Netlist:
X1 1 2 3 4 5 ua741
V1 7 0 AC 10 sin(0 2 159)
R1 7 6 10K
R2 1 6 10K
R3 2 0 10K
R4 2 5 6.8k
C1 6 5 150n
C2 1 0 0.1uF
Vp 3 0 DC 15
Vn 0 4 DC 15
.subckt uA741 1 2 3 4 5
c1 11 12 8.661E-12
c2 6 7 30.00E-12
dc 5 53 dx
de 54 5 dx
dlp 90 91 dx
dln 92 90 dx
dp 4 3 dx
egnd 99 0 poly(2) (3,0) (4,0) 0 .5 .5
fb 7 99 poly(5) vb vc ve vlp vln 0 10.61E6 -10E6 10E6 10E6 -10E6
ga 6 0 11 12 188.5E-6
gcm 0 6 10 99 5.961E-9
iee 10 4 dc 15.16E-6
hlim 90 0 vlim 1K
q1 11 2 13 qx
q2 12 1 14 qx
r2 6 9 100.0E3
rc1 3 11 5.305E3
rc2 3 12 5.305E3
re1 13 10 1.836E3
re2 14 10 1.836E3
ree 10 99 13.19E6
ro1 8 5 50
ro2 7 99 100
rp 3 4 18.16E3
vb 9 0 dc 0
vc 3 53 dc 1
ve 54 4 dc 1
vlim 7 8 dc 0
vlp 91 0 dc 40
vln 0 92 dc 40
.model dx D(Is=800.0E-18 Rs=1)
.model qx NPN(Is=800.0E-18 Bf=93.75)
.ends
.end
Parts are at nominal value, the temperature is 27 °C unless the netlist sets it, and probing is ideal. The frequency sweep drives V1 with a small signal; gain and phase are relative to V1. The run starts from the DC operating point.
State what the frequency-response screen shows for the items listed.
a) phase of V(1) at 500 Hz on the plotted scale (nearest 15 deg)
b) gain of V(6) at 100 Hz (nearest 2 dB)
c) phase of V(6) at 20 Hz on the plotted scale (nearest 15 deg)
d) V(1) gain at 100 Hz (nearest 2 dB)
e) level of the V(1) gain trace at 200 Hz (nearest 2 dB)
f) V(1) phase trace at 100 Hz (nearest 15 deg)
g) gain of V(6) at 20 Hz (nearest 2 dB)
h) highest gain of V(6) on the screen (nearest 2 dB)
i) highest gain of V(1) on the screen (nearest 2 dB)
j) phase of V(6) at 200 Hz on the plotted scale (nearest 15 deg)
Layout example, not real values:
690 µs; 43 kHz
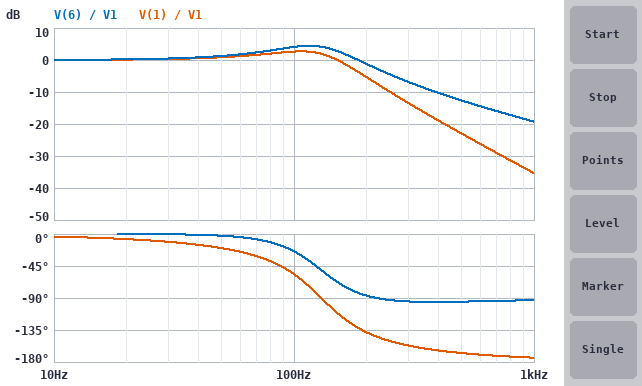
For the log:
-165 deg; 4 dB; 0 deg; 2 dB; -6 dB; -60 deg; 0 dB; 4 dB; 2 dB; -90 deg
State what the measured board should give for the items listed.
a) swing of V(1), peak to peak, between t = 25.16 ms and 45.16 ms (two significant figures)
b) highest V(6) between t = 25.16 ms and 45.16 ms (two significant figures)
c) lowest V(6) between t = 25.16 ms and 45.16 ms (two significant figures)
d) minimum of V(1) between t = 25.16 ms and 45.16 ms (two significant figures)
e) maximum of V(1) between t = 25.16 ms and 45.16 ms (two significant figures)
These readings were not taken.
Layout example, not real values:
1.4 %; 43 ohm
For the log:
3.6 V; 2.6 V; -2.6 V; -1.8 V; 1.8 V
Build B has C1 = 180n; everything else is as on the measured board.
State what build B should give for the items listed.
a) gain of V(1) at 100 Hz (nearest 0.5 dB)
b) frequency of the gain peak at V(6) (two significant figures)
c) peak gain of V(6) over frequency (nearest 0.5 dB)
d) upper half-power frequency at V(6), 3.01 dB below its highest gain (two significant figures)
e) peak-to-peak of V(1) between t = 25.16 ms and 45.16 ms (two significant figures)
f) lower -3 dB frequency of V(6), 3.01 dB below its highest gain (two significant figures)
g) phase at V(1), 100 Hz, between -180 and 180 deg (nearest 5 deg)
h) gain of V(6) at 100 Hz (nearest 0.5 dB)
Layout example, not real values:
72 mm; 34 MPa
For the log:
5.0 dB; 110 Hz; 7.0 dB; 150 Hz; 3.6 V; 74 Hz; -60 deg; 6.5 dB
